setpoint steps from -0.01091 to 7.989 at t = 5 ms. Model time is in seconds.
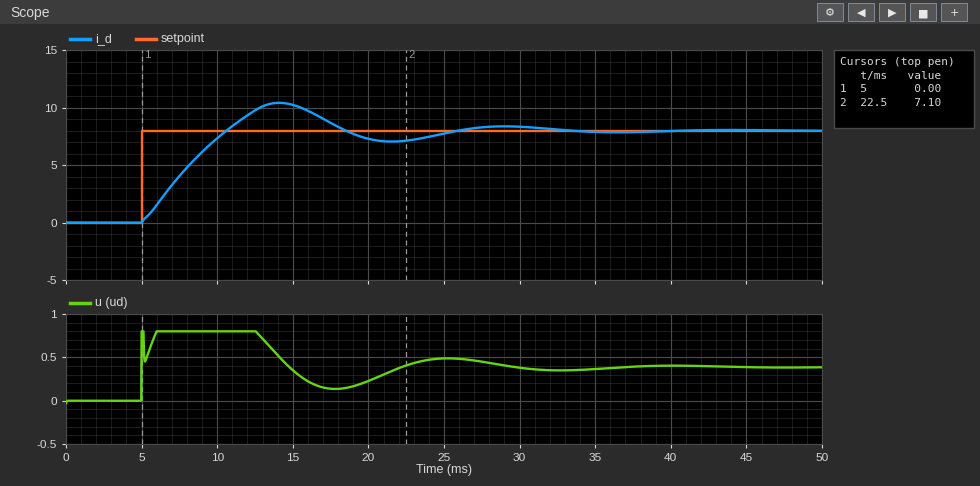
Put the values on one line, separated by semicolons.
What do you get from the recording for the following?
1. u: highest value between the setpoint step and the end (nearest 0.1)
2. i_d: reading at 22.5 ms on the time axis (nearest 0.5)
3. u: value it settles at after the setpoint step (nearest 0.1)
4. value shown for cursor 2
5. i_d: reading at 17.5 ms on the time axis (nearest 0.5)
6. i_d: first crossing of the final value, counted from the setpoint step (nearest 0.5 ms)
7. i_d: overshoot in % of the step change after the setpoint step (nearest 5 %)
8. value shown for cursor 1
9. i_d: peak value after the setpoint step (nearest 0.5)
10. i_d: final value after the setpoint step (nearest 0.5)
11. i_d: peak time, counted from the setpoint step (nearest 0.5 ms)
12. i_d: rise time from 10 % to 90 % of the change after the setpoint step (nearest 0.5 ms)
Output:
0.8; 7.0; 0.4; 7.10; 8.5; 5.5 ms; 30 %; 0.00; 10.5; 8.0; 9.0 ms; 4.5 ms
